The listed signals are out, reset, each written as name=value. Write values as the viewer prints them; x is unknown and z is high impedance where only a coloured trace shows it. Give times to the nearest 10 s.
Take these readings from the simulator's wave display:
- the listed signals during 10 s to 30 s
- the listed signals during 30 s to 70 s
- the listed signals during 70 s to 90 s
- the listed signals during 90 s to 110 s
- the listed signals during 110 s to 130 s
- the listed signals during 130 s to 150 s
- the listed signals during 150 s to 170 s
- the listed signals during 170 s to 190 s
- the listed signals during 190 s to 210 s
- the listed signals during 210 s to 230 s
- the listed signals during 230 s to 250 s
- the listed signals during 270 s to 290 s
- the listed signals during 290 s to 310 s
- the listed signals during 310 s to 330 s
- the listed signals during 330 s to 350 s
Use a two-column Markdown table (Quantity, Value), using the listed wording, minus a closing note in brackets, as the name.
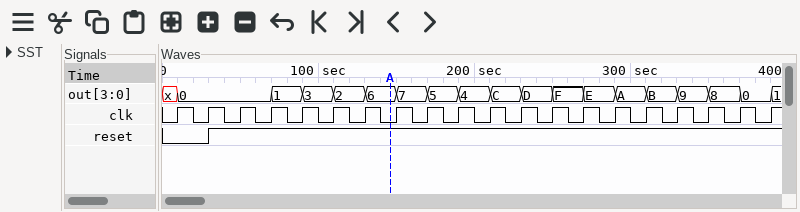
| Quantity | Value |
|---|---|
| the listed signals during 10 s to 30 s | out=0, reset=0 |
| the listed signals during 30 s to 70 s | out=0, reset=1 |
| the listed signals during 70 s to 90 s | out=1, reset=1 |
| the listed signals during 90 s to 110 s | out=3, reset=1 |
| the listed signals during 110 s to 130 s | out=2, reset=1 |
| the listed signals during 130 s to 150 s | out=6, reset=1 |
| the listed signals during 150 s to 170 s | out=7, reset=1 |
| the listed signals during 170 s to 190 s | out=5, reset=1 |
| the listed signals during 190 s to 210 s | out=4, reset=1 |
| the listed signals during 210 s to 230 s | out=C, reset=1 |
| the listed signals during 230 s to 250 s | out=D, reset=1 |
| the listed signals during 270 s to 290 s | out=E, reset=1 |
| the listed signals during 290 s to 310 s | out=A, reset=1 |
| the listed signals during 310 s to 330 s | out=B, reset=1 |
| the listed signals during 330 s to 350 s | out=9, reset=1 |
